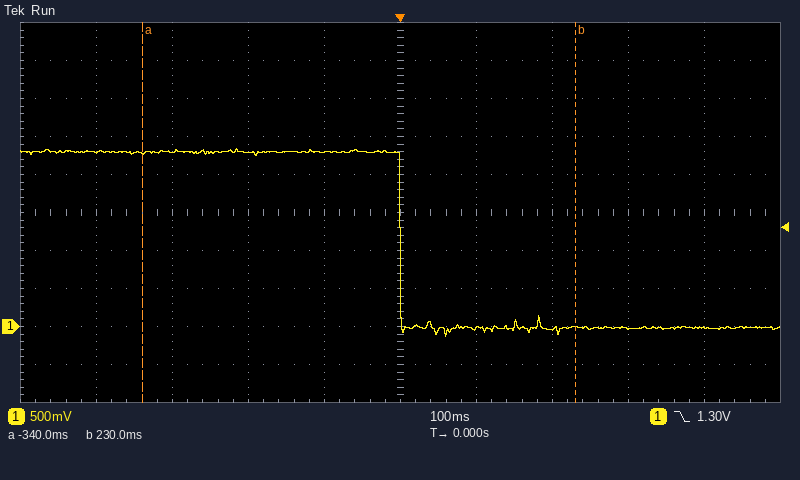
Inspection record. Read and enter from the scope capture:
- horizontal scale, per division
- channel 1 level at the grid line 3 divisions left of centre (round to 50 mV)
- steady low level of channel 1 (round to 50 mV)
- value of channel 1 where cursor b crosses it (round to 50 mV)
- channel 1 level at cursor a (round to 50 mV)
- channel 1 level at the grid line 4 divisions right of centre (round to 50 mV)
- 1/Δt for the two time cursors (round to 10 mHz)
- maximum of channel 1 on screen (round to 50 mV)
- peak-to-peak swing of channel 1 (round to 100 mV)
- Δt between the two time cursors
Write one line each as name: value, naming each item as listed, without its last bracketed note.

horizontal scale, per division: 100 ms
channel 1 level at the grid line 3 divisions left of centre: 2.30 V
steady low level of channel 1: 0 mV
value of channel 1 where cursor b crosses it: 0 mV
channel 1 level at cursor a: 2.30 V
channel 1 level at the grid line 4 divisions right of centre: 0 mV
1/Δt for the two time cursors: 1.75 Hz
maximum of channel 1 on screen: 2.35 V
peak-to-peak swing of channel 1: 2.50 V
Δt between the two time cursors: 570 ms
